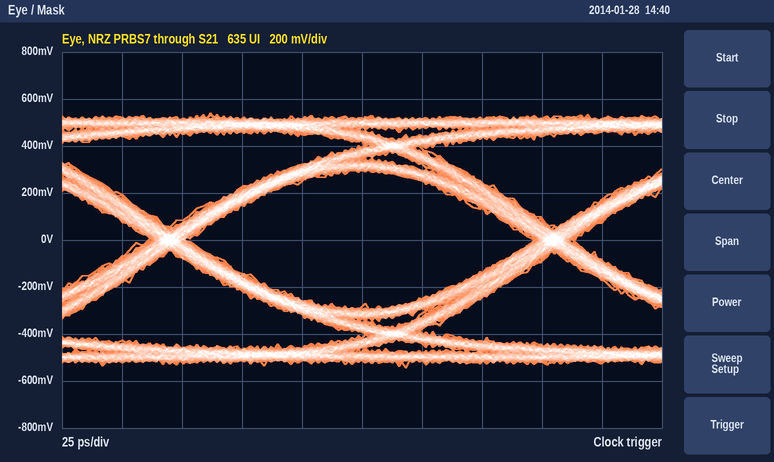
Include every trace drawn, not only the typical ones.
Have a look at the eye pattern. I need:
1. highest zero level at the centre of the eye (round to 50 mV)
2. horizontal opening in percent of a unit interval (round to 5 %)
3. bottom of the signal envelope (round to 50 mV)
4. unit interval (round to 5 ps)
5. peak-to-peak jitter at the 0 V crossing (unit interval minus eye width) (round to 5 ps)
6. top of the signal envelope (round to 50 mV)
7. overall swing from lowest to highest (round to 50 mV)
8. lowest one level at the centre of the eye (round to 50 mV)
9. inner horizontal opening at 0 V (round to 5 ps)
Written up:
-300 mV
90 %
-550 mV
160 ps
15 ps
550 mV
1.10 V
300 mV
145 ps
